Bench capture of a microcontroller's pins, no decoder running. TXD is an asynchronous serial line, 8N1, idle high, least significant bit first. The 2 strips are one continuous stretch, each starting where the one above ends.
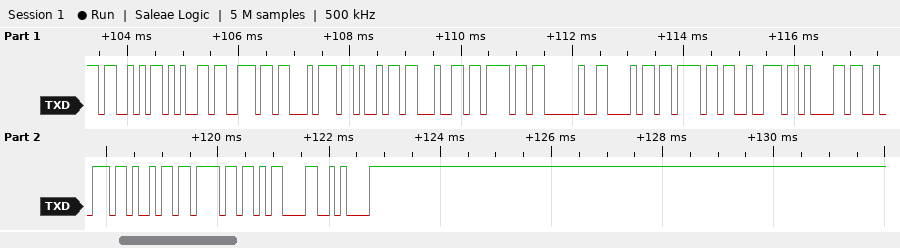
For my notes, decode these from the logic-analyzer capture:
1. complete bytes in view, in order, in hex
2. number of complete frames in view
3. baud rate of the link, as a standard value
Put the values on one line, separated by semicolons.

0x53 0x65 0x6E 0x74 0x69 0x64 0x6F 0x20 0x68 0x6F 0x72 0x61 0x72 0x69 0x6F 0x0D 0x0A; 17; 9600 baud
